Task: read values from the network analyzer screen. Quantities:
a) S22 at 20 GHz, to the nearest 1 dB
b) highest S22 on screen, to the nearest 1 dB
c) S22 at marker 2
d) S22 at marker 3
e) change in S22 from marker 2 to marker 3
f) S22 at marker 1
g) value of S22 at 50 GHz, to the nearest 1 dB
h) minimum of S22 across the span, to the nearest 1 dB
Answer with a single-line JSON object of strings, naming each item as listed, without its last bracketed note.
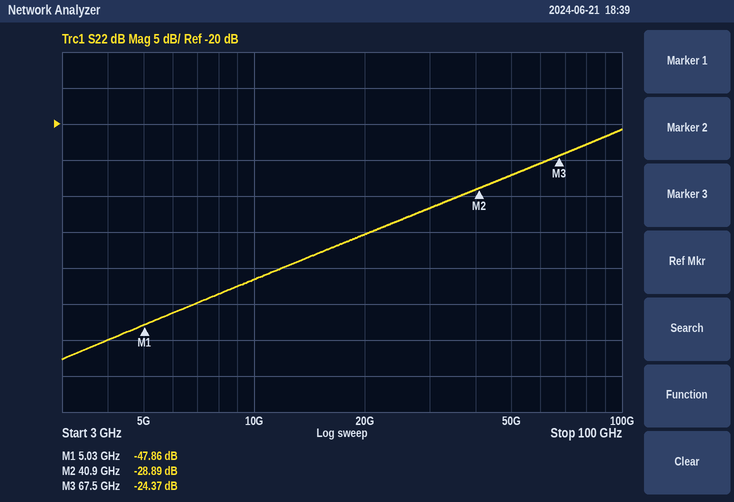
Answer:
{"S22 at 20 GHz, to the nearest 1 dB": "-35 dB", "highest S22 on screen, to the nearest 1 dB": "-21 dB", "S22 at marker 2": "-28.89 dB", "S22 at marker 3": "-24.37 dB", "change in S22 from marker 2 to marker 3": "4.52 dB", "S22 at marker 1": "-47.86 dB", "value of S22 at 50 GHz, to the nearest 1 dB": "-27 dB", "minimum of S22 across the span, to the nearest 1 dB": "-53 dB"}
